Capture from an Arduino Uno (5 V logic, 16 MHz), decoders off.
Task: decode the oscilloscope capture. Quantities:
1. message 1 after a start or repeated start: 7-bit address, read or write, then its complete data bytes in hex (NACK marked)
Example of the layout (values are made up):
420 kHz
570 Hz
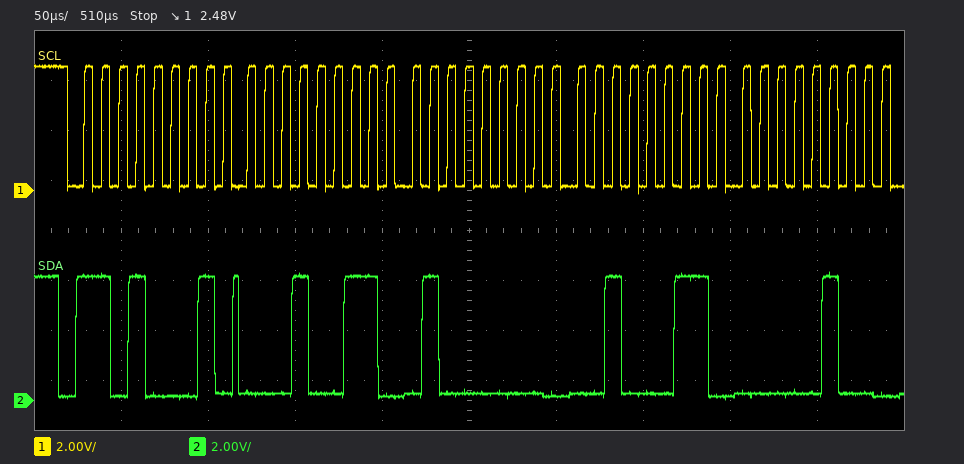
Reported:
0x68 read: 13 40 23 04
